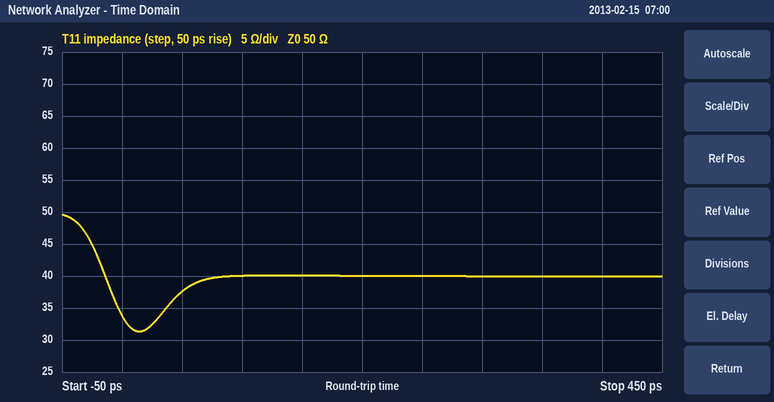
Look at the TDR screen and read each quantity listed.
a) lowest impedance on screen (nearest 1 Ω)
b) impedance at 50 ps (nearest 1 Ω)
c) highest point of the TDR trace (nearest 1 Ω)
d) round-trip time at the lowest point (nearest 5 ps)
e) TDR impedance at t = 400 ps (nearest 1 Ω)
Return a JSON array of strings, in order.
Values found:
["31 Ω", "38 Ω", "50 Ω", "15 ps", "40 Ω"]
